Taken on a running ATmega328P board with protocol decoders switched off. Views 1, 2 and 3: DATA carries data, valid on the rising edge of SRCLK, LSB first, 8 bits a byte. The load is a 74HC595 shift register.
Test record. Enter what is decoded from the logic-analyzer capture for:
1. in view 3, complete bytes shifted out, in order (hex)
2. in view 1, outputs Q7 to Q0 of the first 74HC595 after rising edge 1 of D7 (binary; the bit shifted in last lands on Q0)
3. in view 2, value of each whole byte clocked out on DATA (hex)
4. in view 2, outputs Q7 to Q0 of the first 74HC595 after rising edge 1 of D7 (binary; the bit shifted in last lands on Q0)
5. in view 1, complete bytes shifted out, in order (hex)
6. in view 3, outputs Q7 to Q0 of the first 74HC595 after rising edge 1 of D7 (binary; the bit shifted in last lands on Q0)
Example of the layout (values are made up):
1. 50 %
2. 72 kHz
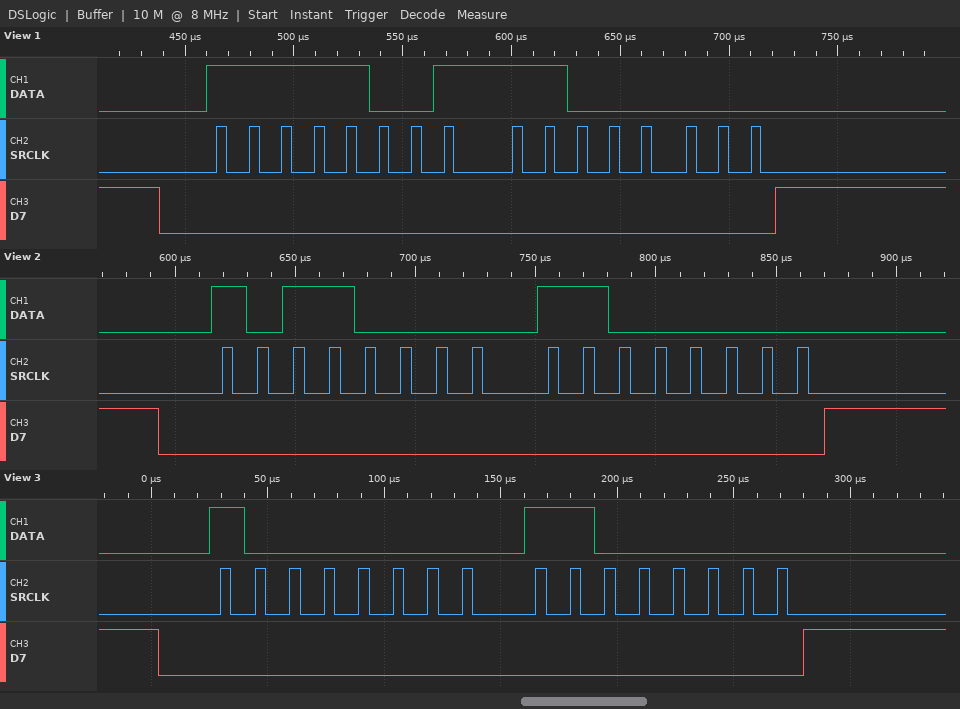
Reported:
1. 01 03
2. 11000000
3. 0x0D 0x03
4. 11000000
5. 9F 03
6. 11000000
